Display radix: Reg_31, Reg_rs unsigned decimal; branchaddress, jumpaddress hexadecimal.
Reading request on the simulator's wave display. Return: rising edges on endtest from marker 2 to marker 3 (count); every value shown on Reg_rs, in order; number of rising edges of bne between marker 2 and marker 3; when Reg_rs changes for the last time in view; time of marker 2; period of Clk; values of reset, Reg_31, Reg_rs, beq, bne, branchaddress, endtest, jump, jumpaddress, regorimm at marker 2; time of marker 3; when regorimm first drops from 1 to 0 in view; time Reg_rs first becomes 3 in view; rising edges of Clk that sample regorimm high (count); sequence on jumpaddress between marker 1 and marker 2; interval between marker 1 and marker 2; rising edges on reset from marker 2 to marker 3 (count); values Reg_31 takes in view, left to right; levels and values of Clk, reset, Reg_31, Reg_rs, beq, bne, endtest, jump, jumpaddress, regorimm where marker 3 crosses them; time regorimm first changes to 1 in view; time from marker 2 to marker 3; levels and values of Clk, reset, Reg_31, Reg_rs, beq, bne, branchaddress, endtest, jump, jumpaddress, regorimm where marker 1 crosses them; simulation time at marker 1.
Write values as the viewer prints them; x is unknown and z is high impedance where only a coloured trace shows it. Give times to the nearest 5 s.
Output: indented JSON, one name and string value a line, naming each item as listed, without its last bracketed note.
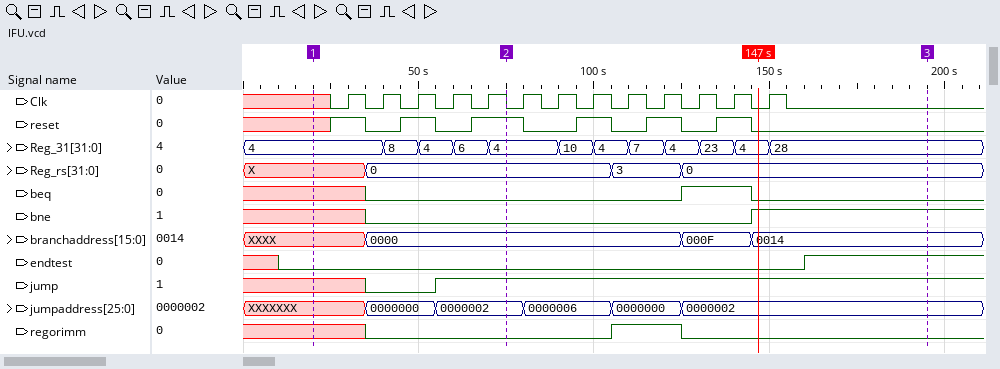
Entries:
{
  "rising edges on endtest from marker 2 to marker 3": "1",
  "every value shown on Reg_rs, in order": "X, 0, 3, 0",
  "number of rising edges of bne between marker 2 and marker 3": "1",
  "when Reg_rs changes for the last time in view": "125 s",
  "time of marker 2": "75 s",
  "period of Clk": "10 s",
  "values of reset, Reg_31, Reg_rs, beq, bne, branchaddress, endtest, jump, jumpaddress, regorimm at marker 2": "reset=1, Reg_31=4, Reg_rs=0, beq=0, bne=0, branchaddress=0000, endtest=0, jump=1, jumpaddress=0000002, regorimm=0",
  "time of marker 3": "195 s",
  "when regorimm first drops from 1 to 0 in view": "125 s",
  "time Reg_rs first becomes 3 in view": "105 s",
  "rising edges of Clk that sample regorimm high": "2",
  "sequence on jumpaddress between marker 1 and marker 2": "XXXXXXX, 0000000, 0000002",
  "interval between marker 1 and marker 2": "55 s",
  "rising edges on reset from marker 2 to marker 3": "3",
  "values Reg_31 takes in view, left to right": "4, 8, 4, 6, 4, 10, 4, 7, 4, 23, 4, 28",
  "levels and values of Clk, reset, Reg_31, Reg_rs, beq, bne, endtest, jump, jumpaddress, regorimm where marker 3 crosses them": "Clk=0, reset=0, Reg_31=28, Reg_rs=0, beq=0, bne=1, endtest=1, jump=1, jumpaddress=0000002, regorimm=0",
  "time regorimm first changes to 1 in view": "105 s",
  "time from marker 2 to marker 3": "120 s",
  "levels and values of Clk, reset, Reg_31, Reg_rs, beq, bne, branchaddress, endtest, jump, jumpaddress, regorimm where marker 1 crosses them": "Clk=x, reset=x, Reg_31=4, Reg_rs=X, beq=x, bne=x, branchaddress=XXXX, endtest=0, jump=x, jumpaddress=XXXXXXX, regorimm=x",
  "simulation time at marker 1": "20 s"
}
